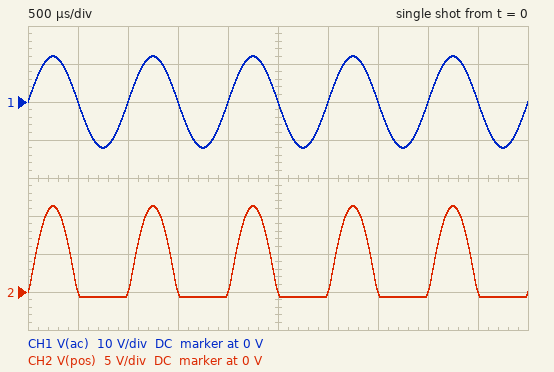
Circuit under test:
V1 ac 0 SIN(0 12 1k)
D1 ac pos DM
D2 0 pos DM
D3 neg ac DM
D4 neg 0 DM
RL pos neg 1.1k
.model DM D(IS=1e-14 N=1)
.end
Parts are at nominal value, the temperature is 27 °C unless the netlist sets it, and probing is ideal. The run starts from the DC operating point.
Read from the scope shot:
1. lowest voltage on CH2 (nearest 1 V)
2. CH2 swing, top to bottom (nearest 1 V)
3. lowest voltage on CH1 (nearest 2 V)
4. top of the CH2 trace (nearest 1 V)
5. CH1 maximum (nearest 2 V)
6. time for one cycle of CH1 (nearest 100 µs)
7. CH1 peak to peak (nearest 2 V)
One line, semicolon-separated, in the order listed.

-1 V; 12 V; -12 V; 11 V; 12 V; 1.0 ms; 24 V
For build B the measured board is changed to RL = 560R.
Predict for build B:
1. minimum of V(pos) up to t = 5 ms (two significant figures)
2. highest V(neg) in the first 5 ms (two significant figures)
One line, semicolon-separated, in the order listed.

-730 mV; 730 mV
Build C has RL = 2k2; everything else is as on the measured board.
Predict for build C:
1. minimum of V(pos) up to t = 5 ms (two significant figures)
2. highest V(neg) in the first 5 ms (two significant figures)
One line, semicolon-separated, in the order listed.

-700 mV; 700 mV
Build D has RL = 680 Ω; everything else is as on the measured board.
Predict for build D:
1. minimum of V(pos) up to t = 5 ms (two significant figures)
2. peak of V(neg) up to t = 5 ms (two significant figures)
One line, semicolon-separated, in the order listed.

-730 mV; 730 mV
